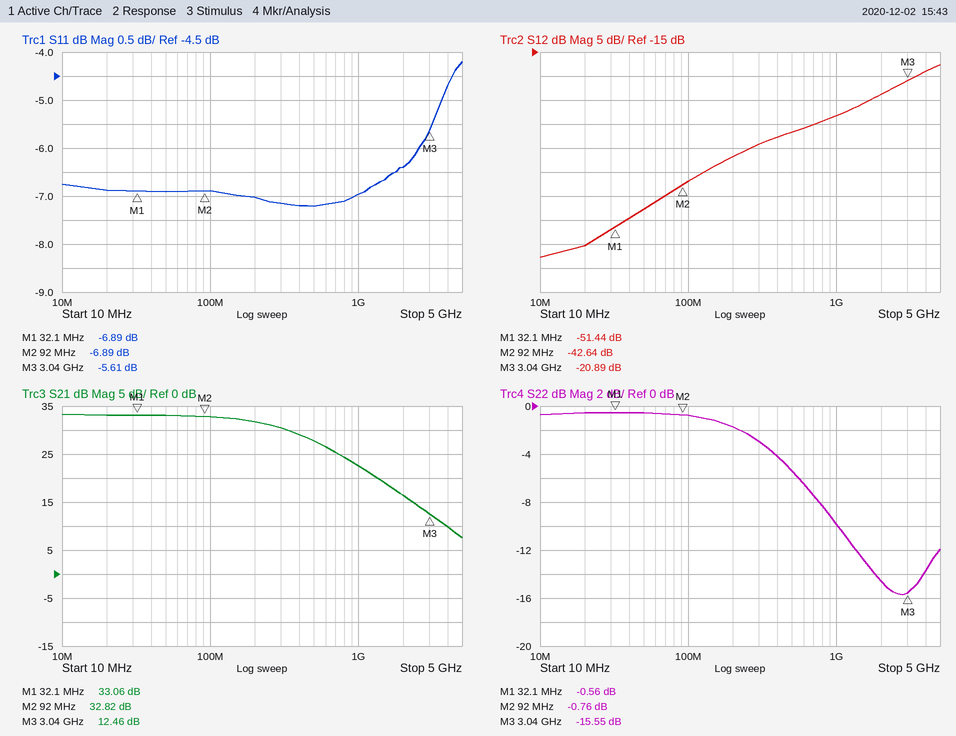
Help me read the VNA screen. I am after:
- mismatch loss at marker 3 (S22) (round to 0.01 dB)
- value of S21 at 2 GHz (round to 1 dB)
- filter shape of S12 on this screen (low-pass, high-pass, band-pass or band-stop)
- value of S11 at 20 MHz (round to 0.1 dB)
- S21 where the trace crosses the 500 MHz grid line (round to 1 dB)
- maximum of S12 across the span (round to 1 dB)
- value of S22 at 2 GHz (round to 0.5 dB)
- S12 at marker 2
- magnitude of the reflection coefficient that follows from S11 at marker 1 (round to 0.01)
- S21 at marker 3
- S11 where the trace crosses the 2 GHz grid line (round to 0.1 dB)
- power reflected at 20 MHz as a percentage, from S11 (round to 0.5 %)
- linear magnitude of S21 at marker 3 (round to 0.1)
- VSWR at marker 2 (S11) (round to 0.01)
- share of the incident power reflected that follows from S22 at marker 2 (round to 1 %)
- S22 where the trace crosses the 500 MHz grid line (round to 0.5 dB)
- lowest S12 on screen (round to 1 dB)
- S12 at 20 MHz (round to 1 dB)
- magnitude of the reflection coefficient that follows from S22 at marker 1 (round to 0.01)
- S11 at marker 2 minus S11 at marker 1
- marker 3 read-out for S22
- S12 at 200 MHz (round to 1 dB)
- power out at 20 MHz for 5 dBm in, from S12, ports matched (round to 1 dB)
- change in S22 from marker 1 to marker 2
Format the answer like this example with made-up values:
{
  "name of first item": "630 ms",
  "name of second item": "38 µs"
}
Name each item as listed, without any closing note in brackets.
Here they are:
{
  "mismatch loss at marker 3 (S22)": "0.12 dB",
  "value of S21 at 2 GHz": "16 dB",
  "filter shape of S12 on this screen": "high-pass",
  "value of S11 at 20 MHz": "-6.9 dB",
  "S21 where the trace crosses the 500 MHz grid line": "28 dB",
  "maximum of S12 across the span": "-18 dB",
  "value of S22 at 2 GHz": "-14.5 dB",
  "S12 at marker 2": "-42.64 dB",
  "magnitude of the reflection coefficient that follows from S11 at marker 1": "0.45",
  "S21 at marker 3": "12.46 dB",
  "S11 where the trace crosses the 2 GHz grid line": "-6.4 dB",
  "power reflected at 20 MHz as a percentage, from S11": "20.5 %",
  "linear magnitude of S21 at marker 3": "4.2",
  "VSWR at marker 2 (S11)": "2.65",
  "share of the incident power reflected that follows from S22 at marker 2": "84 %",
  "S22 where the trace crosses the 500 MHz grid line": "-5.5 dB",
  "lowest S12 on screen": "-58 dB",
  "S12 at 20 MHz": "-55 dB",
  "magnitude of the reflection coefficient that follows from S22 at marker 1": "0.94",
  "S11 at marker 2 minus S11 at marker 1": "0.00 dB",
  "marker 3 read-out for S22": "-15.55 dB",
  "S12 at 200 MHz": "-37 dB",
  "power out at 20 MHz for 5 dBm in, from S12, ports matched": "-50 dBm",
  "change in S22 from marker 1 to marker 2": "-0.20 dB"
}
